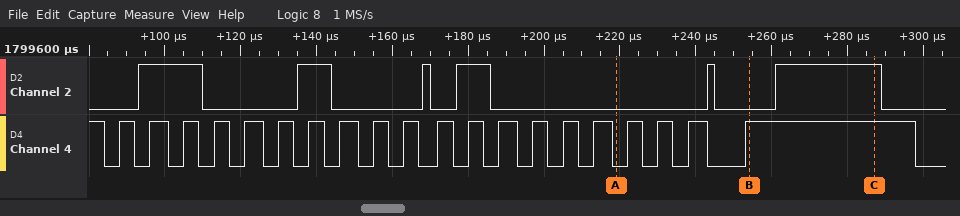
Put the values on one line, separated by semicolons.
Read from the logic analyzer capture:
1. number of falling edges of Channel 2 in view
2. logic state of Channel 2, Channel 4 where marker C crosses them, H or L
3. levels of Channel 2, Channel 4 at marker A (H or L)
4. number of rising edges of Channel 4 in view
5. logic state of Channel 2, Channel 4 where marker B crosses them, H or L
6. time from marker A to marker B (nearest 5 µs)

6; Channel 2=H, Channel 4=H; Channel 2=L, Channel 4=L; 20; Channel 2=L, Channel 4=H; 35 µs
